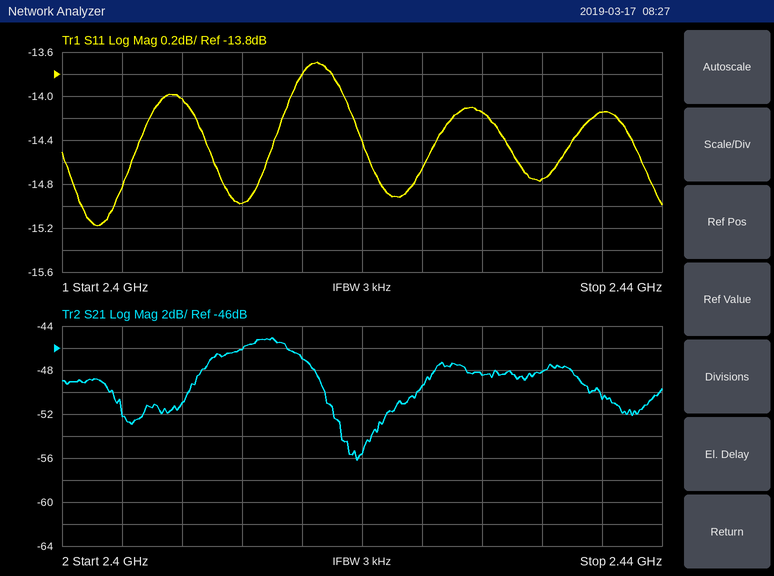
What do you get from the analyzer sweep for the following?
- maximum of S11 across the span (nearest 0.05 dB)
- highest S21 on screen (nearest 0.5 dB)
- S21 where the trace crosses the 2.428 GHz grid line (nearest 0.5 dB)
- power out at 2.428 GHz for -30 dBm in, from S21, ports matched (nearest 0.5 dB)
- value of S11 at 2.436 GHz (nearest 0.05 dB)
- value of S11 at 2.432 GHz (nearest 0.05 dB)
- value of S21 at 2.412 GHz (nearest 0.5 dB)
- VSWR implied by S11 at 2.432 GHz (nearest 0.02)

-13.70 dB
-45.0 dB
-48.5 dB
-78.5 dBm
-14.15 dB
-14.75 dB
-46.0 dB
1.44
